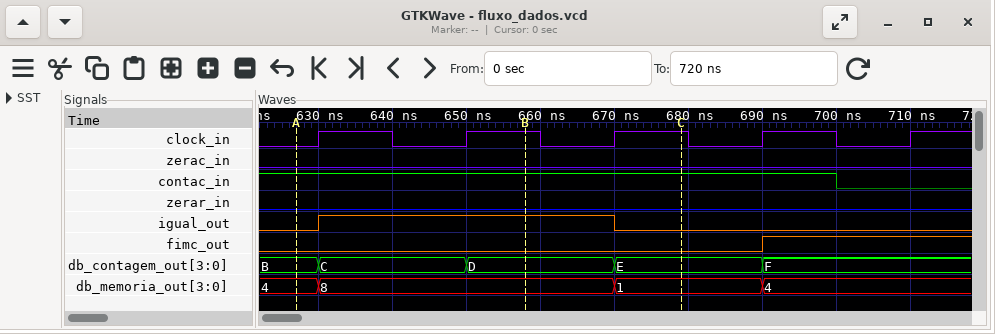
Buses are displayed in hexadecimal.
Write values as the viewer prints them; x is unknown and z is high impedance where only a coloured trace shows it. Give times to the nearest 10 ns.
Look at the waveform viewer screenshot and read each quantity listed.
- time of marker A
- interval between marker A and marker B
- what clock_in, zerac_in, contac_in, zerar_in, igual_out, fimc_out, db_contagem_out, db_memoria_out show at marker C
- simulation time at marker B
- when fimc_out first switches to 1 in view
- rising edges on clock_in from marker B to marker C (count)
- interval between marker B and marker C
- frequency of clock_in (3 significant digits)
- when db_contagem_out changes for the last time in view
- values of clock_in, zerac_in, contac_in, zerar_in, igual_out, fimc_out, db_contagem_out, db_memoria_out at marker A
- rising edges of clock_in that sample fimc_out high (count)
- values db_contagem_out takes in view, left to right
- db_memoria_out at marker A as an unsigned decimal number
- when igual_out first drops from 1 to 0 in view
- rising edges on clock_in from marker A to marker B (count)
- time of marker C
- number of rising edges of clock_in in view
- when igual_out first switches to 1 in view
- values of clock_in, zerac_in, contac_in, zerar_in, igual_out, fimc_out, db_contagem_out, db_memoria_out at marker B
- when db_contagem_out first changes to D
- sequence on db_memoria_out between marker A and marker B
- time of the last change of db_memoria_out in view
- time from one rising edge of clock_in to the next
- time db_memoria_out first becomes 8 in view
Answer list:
630 ns
30 ns
clock_in=1, zerac_in=0, contac_in=1, zerar_in=0, igual_out=0, fimc_out=0, db_contagem_out=E, db_memoria_out=1
660 ns
690 ns
1
20 ns
50.0 MHz
690 ns
clock_in=0, zerac_in=0, contac_in=1, zerar_in=0, igual_out=0, fimc_out=0, db_contagem_out=B, db_memoria_out=4
1
B, C, D, E, F
4
670 ns
2
680 ns
5
630 ns
clock_in=1, zerac_in=0, contac_in=1, zerar_in=0, igual_out=1, fimc_out=0, db_contagem_out=D, db_memoria_out=8
650 ns
4, 8
690 ns
20 ns
630 ns
